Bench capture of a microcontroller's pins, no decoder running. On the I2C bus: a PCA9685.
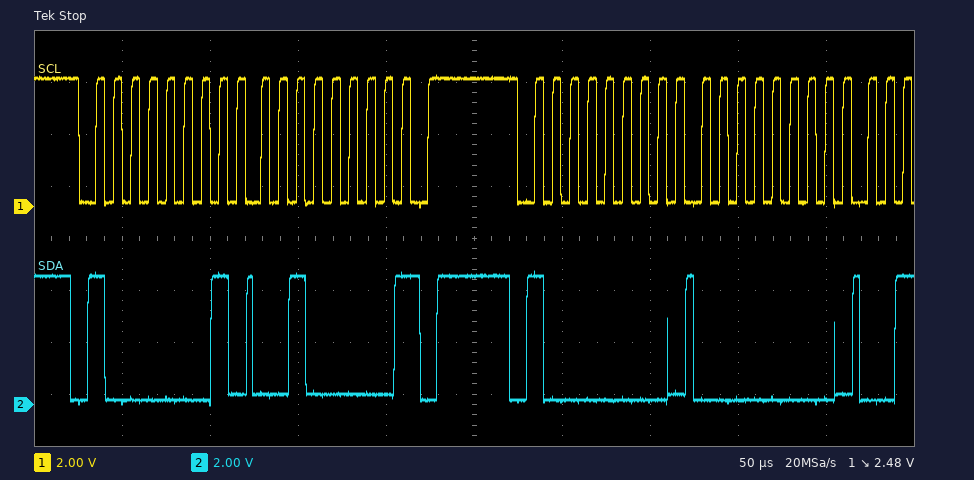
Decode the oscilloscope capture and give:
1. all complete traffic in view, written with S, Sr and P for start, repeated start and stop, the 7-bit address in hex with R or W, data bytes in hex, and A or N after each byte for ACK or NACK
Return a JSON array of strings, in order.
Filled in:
["S 40R A 20 N P S 40W A 00 A"]
